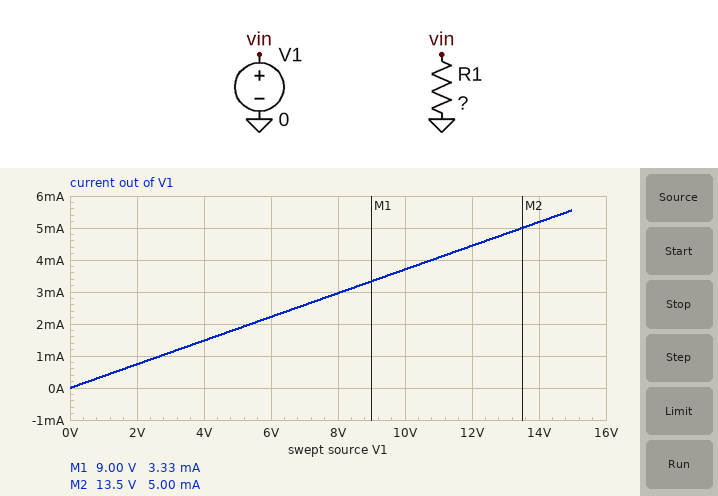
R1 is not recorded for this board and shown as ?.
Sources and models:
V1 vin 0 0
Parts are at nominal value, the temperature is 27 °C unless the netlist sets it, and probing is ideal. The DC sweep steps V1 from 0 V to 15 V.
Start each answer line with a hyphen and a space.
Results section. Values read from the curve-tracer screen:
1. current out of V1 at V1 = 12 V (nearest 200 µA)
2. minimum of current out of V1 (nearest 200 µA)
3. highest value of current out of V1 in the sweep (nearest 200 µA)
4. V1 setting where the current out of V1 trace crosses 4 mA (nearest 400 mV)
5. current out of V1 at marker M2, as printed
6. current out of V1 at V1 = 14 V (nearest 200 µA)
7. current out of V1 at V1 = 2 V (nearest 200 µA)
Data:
- 4.4 mA
- 0 A
- 5.6 mA
- 10.8 V
- 5.00 mA
- 5.2 mA
- 800 µA
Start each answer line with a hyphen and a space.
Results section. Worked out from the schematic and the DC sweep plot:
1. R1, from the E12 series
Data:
- 2.7 kΩ
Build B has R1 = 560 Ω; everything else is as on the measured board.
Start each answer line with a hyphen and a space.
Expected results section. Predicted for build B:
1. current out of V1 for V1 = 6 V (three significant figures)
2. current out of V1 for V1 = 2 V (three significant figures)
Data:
- 10.7 mA
- 3.57 mA
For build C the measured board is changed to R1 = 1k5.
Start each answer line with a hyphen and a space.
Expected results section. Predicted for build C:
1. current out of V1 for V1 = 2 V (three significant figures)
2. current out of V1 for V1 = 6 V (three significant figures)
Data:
- 1.33 mA
- 4.00 mA
